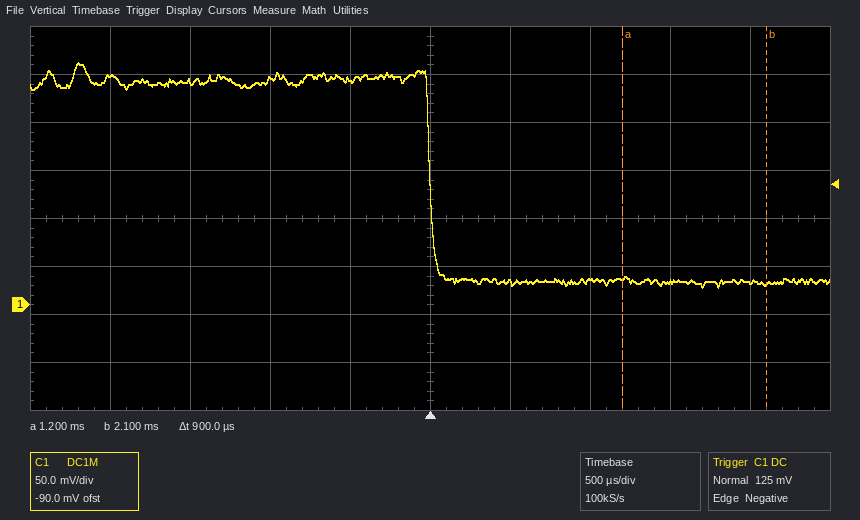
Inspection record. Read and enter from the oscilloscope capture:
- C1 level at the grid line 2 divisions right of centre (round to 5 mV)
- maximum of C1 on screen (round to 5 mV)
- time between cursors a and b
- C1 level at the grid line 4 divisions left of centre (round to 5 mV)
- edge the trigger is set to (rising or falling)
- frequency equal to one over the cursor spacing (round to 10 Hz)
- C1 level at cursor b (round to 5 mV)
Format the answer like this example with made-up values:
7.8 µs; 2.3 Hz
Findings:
25 mV; 250 mV; 900 µs; 240 mV; falling; 1.11 kHz; 20 mV
